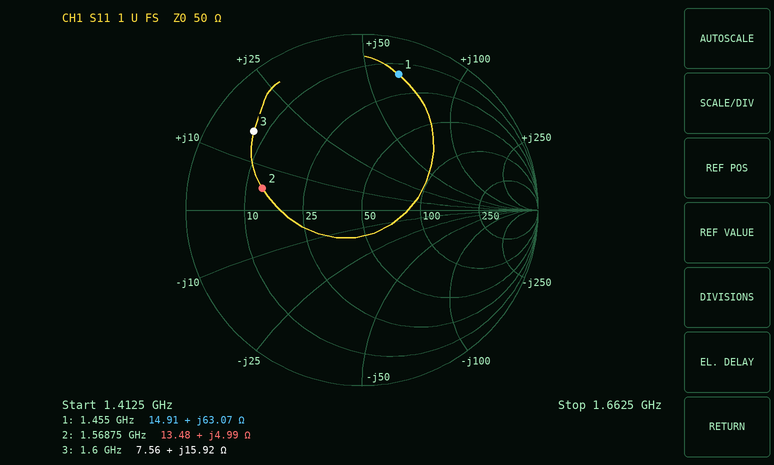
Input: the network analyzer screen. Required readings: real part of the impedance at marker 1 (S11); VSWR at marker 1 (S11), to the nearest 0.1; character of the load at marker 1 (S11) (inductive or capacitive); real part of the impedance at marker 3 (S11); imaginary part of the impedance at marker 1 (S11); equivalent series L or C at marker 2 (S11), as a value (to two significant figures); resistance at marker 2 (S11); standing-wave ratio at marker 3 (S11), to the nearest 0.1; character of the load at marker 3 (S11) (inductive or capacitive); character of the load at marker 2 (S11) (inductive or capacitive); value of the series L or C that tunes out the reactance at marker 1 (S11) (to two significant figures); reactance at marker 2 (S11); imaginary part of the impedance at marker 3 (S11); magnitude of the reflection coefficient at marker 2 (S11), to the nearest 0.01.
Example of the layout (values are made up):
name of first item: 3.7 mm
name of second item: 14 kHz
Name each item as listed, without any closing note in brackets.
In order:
real part of the impedance at marker 1: 14.91 Ω
VSWR at marker 1 (S11), to the nearest 0.1: 8.9
character of the load at marker 1 (S11): inductive
real part of the impedance at marker 3: 7.56 Ω
imaginary part of the impedance at marker 1: +63.07 Ω
equivalent series L or C at marker 2 (S11), as a value: 510 pH
resistance at marker 2: 13.48 Ω
standing-wave ratio at marker 3 (S11), to the nearest 0.1: 7.3
character of the load at marker 3 (S11): inductive
character of the load at marker 2 (S11): inductive
value of the series L or C that tunes out the reactance at marker 1 (S11): 1.7 pF
reactance at marker 2: +4.99 Ω
imaginary part of the impedance at marker 3: +15.92 Ω
magnitude of the reflection coefficient at marker 2 (S11), to the nearest 0.01: 0.58
